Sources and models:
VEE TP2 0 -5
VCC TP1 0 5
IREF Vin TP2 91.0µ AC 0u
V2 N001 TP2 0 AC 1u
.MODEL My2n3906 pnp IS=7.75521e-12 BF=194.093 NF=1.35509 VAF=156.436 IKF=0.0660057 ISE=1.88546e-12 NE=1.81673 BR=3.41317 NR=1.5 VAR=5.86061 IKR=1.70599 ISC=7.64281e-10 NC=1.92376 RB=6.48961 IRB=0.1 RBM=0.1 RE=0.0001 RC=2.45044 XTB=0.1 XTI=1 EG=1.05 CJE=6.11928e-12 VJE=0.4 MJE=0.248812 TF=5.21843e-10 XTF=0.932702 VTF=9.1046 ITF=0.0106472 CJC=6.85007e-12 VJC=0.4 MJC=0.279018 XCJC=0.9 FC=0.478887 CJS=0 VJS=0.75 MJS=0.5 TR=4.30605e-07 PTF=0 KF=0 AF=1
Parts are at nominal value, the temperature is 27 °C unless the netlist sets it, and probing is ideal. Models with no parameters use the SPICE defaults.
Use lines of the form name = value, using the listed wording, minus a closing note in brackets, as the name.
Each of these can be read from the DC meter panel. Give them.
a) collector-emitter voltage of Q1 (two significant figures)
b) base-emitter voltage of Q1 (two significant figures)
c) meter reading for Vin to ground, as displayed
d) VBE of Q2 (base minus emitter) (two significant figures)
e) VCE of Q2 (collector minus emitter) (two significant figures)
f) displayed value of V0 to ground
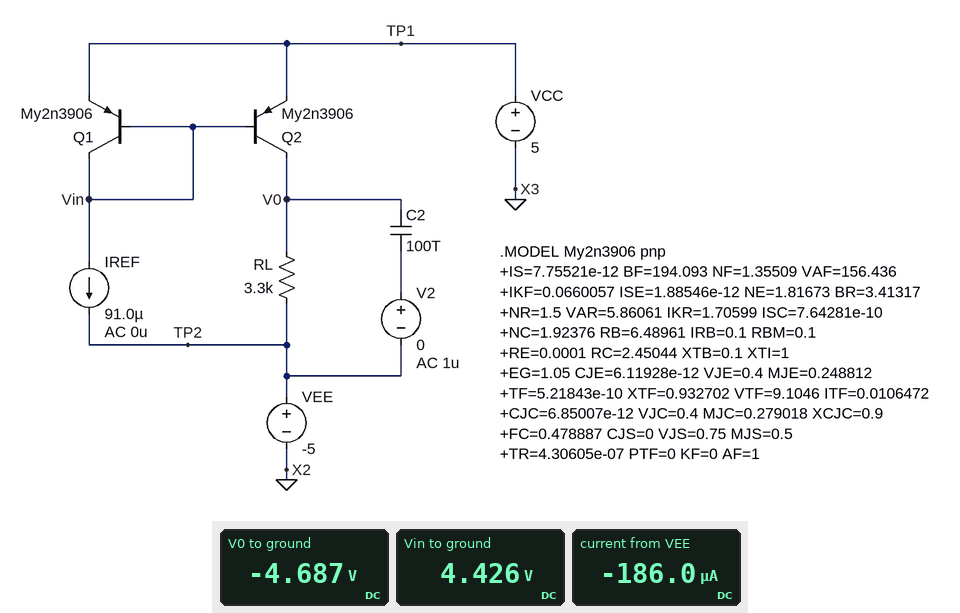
collector-emitter voltage of Q1 = -570 mV
base-emitter voltage of Q1 = -570 mV
meter reading for Vin to ground, as displayed = 4.426 V
VBE of Q2 (base minus emitter) = -570 mV
VCE of Q2 (collector minus emitter) = -9.7 V
displayed value of V0 to ground = -4.687 V
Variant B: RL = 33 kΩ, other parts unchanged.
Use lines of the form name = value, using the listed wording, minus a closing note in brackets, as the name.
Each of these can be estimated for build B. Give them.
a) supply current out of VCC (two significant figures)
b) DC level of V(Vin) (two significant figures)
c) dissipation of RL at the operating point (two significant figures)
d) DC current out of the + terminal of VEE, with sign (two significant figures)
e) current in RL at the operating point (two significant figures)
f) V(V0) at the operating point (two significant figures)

supply current out of VCC = 180 µA
DC level of V(Vin) = 4.4 V
dissipation of RL at the operating point = 290 µW
DC current out of the + terminal of VEE, with sign = -180 µA
current in RL at the operating point = 93 µA
V(V0) at the operating point = -1.9 V
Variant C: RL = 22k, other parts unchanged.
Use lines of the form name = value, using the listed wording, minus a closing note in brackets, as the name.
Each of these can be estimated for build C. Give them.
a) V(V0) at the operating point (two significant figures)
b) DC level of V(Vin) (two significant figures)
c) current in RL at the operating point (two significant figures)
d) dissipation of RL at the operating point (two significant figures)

V(V0) at the operating point = -2.9 V
DC level of V(Vin) = 4.4 V
current in RL at the operating point = 94 µA
dissipation of RL at the operating point = 190 µW
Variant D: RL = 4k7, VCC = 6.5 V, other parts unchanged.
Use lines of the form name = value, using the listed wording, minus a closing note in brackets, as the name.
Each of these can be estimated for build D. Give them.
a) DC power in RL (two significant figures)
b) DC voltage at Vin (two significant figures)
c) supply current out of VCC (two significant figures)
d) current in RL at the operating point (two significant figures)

DC power in RL = 43 µW
DC voltage at Vin = 5.9 V
supply current out of VCC = 190 µA
current in RL at the operating point = 96 µA
